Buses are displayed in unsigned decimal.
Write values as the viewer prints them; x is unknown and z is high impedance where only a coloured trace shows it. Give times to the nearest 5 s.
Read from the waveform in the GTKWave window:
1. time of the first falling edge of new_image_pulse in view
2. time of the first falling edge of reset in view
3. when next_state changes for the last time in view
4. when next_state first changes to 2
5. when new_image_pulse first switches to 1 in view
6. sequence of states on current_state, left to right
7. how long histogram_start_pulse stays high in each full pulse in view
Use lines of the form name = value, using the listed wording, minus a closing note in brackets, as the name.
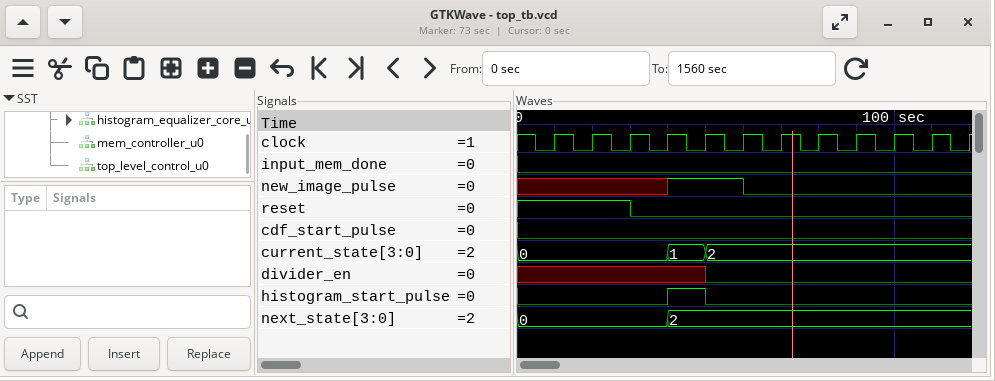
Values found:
time of the first falling edge of new_image_pulse in view = 60 s
time of the first falling edge of reset in view = 30 s
when next_state changes for the last time in view = 40 s
when next_state first changes to 2 = 40 s
when new_image_pulse first switches to 1 in view = 40 s
sequence of states on current_state, left to right = 0, 1, 2
how long histogram_start_pulse stays high in each full pulse in view = 10 s
